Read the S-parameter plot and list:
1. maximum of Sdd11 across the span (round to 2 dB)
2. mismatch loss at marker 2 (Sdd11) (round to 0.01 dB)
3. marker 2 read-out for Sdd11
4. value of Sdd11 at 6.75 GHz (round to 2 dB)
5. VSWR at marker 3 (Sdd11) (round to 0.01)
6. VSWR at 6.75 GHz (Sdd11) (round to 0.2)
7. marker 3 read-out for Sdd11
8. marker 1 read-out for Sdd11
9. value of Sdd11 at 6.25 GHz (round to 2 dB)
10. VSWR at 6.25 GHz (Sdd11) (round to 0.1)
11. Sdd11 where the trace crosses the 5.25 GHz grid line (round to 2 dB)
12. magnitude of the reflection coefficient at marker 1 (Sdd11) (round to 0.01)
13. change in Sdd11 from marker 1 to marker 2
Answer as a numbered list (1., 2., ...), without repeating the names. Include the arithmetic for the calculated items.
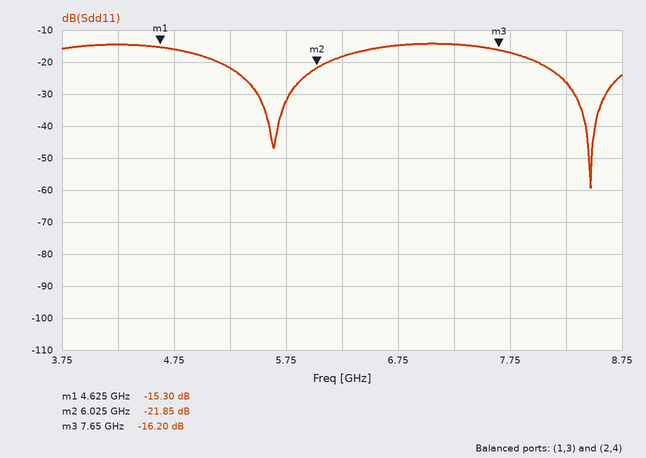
1. -14 dB
2. −10 log10(1 − 10^(-21.85/10)) ≈ 0.03 dB
3. -21.85 dB
4. -14 dB
5. (1 + 0.1549)/(1 − 0.1549) ≈ 1.37
6. |Γ| = 10^(-14/20) = 0.1995; VSWR = (1 + 0.1995)/(1 − 0.1995) ≈ 1.50, so 1.4 to the nearest 0.2
7. -16.20 dB
8. -15.30 dB
9. -18 dB
10. |Γ| = 10^(-18/20) = 0.1259; VSWR = (1 + 0.1259)/(1 − 0.1259) ≈ 1.3
11. -22 dB
12. 10^(-15.3/20) ≈ 0.17
13. -21.85 − (-15.3) = -6.55 dB
